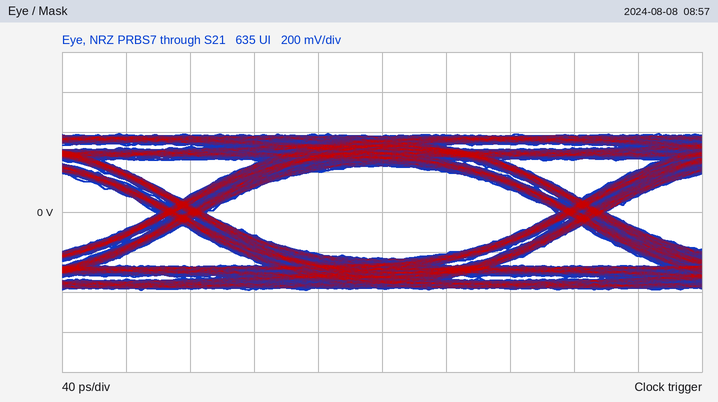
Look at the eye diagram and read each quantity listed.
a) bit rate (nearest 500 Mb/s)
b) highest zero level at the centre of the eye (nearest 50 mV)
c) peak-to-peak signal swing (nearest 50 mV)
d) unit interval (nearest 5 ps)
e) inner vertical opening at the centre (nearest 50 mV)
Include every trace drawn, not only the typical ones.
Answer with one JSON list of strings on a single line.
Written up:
["4.0 Gb/s", "-250 mV", "800 mV", "250 ps", "450 mV"]
